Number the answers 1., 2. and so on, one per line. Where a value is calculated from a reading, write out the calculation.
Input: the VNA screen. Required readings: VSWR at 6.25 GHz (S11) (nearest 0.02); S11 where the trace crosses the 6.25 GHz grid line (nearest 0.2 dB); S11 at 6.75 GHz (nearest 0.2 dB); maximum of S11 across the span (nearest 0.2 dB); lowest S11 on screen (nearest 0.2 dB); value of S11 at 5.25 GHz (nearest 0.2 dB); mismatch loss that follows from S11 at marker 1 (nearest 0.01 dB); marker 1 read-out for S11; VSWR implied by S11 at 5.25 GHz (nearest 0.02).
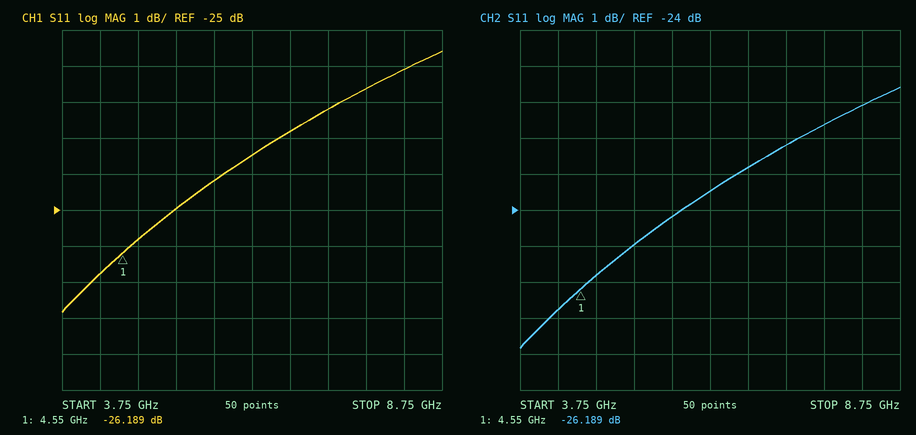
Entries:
1. |Γ| = 10^(-23.4/20) = 0.0676; VSWR = (1 + 0.0676)/(1 − 0.0676) ≈ 1.15, so 1.14 to the nearest 0.02
2. -23.4 dB
3. -22.8 dB
4. -20.6 dB
5. -27.8 dB
6. -25.0 dB
7. −10 log10(1 − 10^(-26.189/10)) ≈ 0.01 dB
8. -26.189 dB
9. |Γ| = 10^(-25/20) = 0.0562; VSWR = (1 + 0.0562)/(1 − 0.0562) ≈ 1.12
